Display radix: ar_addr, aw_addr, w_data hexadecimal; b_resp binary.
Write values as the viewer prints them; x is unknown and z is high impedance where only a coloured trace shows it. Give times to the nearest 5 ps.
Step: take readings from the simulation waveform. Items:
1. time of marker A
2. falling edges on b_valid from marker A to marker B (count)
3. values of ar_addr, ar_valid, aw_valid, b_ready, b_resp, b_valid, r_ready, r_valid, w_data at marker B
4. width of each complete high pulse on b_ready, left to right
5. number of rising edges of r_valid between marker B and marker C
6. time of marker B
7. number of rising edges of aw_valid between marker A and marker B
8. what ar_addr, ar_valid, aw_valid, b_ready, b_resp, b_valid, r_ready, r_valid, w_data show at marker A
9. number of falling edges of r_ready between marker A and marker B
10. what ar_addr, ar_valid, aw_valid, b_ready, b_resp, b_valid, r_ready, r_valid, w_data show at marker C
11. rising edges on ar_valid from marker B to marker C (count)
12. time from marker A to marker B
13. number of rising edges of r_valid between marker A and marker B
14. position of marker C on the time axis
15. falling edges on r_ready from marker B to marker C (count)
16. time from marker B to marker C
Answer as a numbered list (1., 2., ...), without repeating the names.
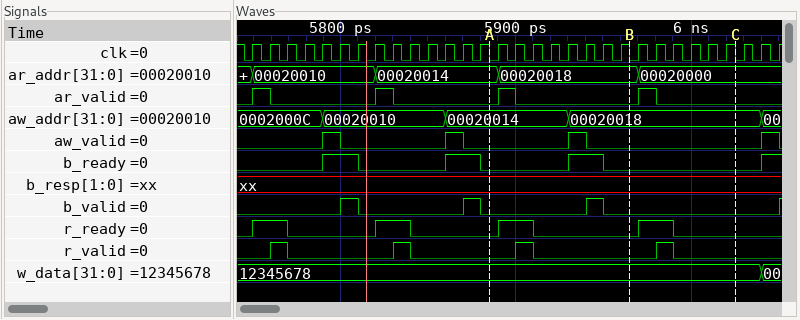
1. 5885 ps
2. 1
3. ar_addr=00020018, ar_valid=0, aw_valid=0, b_ready=0, b_resp=xx, b_valid=0, r_ready=0, r_valid=0, w_data=12345678
4. 20 ps, 20 ps, 20 ps
5. 1
6. 5965 ps
7. 1
8. ar_addr=00020014, ar_valid=0, aw_valid=0, b_ready=0, b_resp=xx, b_valid=0, r_ready=0, r_valid=0, w_data=12345678
9. 1
10. ar_addr=00020000, ar_valid=0, aw_valid=0, b_ready=0, b_resp=xx, b_valid=0, r_ready=0, r_valid=0, w_data=12345678
11. 1
12. 80 ps
13. 1
14. 6025 ps
15. 1
16. 60 ps
